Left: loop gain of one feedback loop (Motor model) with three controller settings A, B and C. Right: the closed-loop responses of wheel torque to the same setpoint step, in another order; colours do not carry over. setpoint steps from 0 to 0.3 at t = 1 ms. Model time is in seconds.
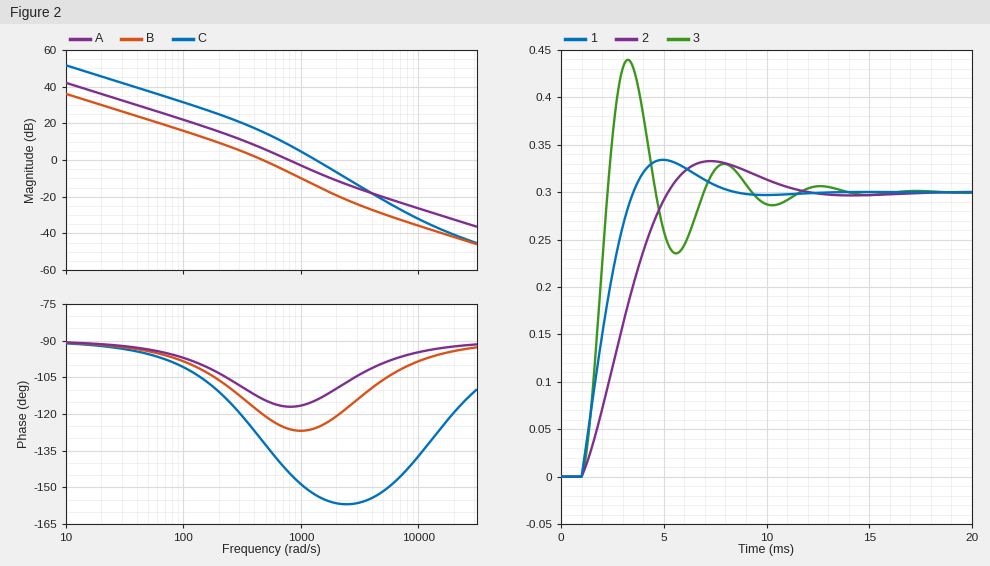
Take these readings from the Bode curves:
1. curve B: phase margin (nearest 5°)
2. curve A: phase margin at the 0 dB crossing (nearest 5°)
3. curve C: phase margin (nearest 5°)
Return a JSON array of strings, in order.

["60°", "65°", "25°"]
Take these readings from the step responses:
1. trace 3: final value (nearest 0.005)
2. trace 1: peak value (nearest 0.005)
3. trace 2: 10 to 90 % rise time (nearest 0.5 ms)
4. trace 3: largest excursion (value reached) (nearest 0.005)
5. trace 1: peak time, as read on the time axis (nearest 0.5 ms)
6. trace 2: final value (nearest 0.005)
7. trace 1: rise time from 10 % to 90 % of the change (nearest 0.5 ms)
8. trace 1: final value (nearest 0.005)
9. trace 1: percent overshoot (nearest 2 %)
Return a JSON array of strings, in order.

["0.300", "0.335", "3.0 ms", "0.440", "5.0 ms", "0.300", "2.0 ms", "0.300", "12 %"]
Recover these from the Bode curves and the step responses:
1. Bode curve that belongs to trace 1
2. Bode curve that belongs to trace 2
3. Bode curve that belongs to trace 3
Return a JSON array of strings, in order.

["A", "B", "C"]
